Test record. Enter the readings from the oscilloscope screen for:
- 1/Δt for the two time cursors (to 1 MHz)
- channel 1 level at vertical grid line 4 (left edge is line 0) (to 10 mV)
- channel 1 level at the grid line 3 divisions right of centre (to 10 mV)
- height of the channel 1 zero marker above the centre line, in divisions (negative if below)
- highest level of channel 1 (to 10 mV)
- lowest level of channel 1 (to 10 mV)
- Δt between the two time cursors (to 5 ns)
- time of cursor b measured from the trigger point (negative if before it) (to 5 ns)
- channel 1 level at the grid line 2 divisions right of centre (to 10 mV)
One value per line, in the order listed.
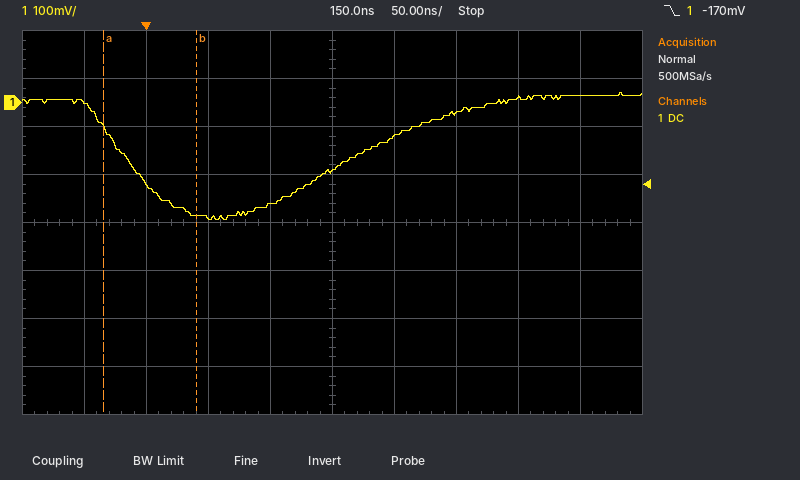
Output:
13 MHz
-210 mV
10 mV
+2.5 div
20 mV
-240 mV
75 ns
+40 ns
-20 mV
